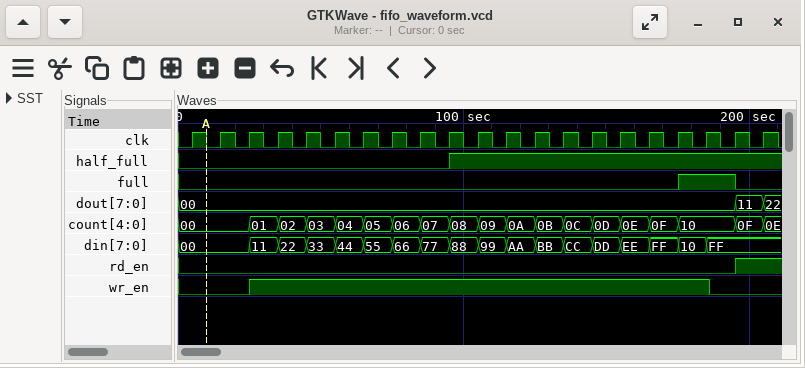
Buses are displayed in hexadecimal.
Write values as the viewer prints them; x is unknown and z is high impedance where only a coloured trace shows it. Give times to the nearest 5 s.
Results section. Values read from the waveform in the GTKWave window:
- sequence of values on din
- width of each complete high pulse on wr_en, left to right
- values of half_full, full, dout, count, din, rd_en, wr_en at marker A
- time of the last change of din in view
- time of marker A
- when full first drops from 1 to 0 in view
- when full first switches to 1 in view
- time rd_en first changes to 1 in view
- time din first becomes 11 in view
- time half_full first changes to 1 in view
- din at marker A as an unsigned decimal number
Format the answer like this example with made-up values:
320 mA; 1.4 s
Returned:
00, 11, 22, 33, 44, 55, 66, 77, 88, 99, AA, BB, CC, DD, EE, FF, 10, FF; 160 s; half_full=0, full=0, dout=00, count=00, din=00, rd_en=0, wr_en=0; 185 s; 10 s; 195 s; 175 s; 195 s; 25 s; 95 s; 0
